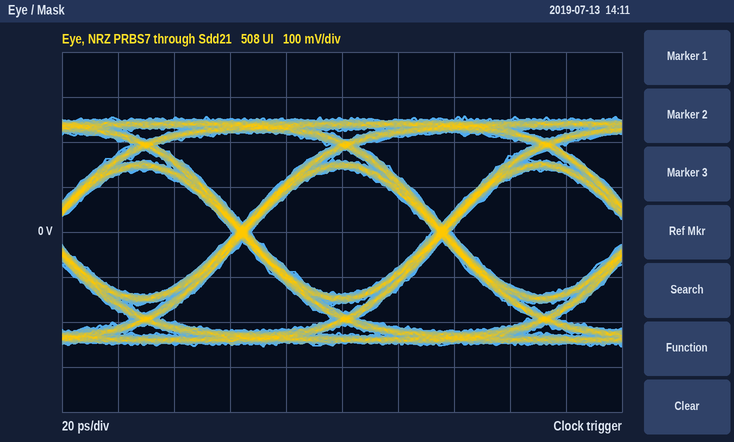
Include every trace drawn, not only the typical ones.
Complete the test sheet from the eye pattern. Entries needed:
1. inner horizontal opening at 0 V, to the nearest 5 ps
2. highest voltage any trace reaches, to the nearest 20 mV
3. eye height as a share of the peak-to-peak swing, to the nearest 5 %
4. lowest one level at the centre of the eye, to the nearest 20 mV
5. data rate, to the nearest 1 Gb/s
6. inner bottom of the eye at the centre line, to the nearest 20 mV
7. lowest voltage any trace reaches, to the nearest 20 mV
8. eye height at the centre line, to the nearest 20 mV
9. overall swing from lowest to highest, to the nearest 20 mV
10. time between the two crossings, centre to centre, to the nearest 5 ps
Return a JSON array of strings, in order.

["65 ps", "260 mV", "55 %", "140 mV", "14 Gb/s", "-140 mV", "-260 mV", "280 mV", "520 mV", "70 ps"]
